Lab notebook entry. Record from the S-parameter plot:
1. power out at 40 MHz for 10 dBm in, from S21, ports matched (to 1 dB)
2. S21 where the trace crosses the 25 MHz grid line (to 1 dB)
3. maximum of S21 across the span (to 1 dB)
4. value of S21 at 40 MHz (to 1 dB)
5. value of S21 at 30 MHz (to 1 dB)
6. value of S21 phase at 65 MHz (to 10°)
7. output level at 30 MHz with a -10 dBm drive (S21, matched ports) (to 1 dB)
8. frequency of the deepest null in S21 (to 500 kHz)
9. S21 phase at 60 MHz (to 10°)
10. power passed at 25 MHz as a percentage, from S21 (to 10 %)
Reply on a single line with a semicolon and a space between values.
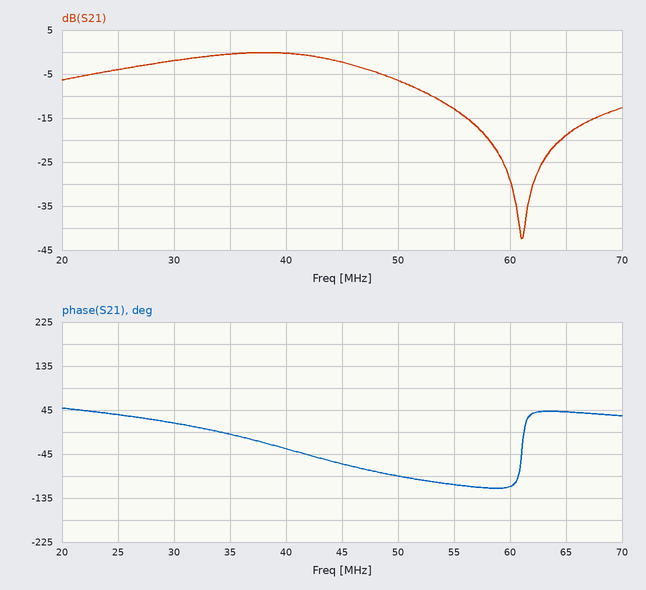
10 dBm; -4 dB; 0 dB; 0 dB; -2 dB; 40°; -12 dBm; 61.0 MHz; -110°; 40 %
